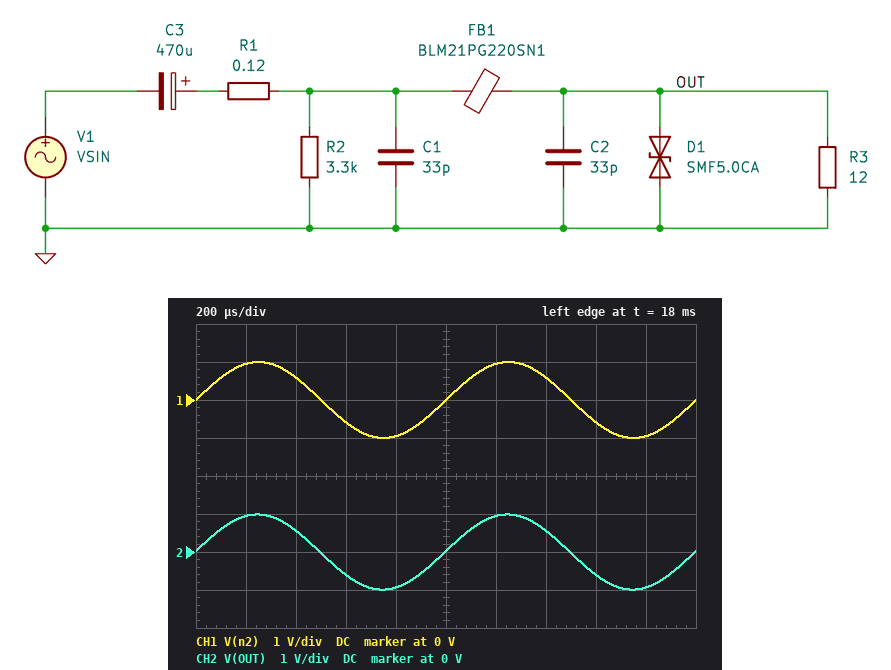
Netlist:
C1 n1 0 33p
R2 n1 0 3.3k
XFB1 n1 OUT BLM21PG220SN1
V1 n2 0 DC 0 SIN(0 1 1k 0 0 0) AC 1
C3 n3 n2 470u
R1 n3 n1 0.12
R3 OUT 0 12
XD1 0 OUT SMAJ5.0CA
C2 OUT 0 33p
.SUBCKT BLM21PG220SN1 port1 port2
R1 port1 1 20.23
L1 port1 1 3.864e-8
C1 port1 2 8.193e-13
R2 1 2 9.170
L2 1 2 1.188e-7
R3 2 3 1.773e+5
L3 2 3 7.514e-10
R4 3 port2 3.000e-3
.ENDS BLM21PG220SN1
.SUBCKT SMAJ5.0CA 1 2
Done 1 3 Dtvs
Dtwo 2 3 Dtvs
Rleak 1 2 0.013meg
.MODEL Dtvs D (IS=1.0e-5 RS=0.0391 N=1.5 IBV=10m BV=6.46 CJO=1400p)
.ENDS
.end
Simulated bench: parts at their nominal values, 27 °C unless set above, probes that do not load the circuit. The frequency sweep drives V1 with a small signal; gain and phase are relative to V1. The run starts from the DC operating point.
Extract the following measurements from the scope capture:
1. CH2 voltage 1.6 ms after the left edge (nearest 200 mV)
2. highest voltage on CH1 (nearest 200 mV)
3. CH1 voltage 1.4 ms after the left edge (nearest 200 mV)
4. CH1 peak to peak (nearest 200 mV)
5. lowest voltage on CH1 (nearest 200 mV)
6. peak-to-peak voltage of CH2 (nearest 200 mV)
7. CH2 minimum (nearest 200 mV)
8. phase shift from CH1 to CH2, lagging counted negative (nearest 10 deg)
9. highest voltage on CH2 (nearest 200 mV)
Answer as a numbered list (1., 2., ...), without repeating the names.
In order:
1. -600 mV
2. 1.0 V
3. 600 mV
4. 2.0 V
5. -1.0 V
6. 2.0 V
7. -1.0 V
8. 0 deg
9. 1.0 V
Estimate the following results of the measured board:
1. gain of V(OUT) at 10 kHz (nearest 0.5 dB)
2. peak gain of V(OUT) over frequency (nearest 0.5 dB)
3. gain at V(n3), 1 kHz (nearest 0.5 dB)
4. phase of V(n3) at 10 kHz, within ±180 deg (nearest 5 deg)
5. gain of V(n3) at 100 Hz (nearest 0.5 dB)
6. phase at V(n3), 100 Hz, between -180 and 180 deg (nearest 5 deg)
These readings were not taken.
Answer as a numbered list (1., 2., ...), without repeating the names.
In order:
1. 0 dB
2. 0 dB
3. 0 dB
4. 0 deg
5. -0.5 dB
6. 15 deg
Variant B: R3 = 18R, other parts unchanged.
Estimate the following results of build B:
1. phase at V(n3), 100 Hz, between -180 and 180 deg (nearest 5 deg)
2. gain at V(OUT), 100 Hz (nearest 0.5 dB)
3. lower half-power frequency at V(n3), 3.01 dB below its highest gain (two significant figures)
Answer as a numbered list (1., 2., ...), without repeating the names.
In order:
1. 10 deg
2. 0 dB
3. 19 Hz
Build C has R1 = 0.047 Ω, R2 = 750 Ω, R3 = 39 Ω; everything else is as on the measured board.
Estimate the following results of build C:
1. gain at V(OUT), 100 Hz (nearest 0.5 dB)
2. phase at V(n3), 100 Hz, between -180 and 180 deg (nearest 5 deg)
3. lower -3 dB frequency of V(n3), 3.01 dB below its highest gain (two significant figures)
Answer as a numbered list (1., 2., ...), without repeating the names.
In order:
1. 0 dB
2. 5 deg
3. 9.2 Hz
